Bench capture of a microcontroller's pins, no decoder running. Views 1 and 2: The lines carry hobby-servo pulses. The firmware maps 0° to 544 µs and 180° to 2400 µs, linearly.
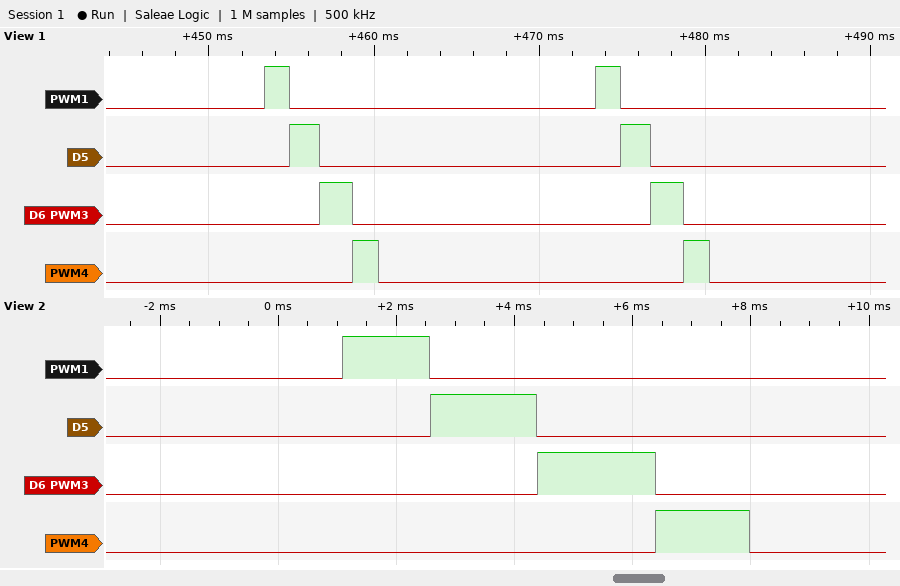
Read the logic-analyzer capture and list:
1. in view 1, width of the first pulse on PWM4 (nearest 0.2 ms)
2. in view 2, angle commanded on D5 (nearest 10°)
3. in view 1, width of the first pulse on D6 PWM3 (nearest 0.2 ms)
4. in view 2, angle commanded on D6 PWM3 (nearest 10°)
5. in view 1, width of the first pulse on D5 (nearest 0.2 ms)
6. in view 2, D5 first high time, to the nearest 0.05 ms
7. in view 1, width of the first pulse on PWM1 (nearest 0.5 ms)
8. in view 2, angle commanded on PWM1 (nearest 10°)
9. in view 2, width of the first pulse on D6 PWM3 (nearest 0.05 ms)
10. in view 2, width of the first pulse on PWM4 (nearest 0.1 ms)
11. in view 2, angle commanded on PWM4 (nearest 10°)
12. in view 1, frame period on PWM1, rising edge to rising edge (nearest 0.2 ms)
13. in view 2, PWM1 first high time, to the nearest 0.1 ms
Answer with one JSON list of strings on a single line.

["1.6 ms", "120°", "2.0 ms", "140°", "1.8 ms", "1.80 ms", "1.5 ms", "90°", "2.00 ms", "1.6 ms", "100°", "20.0 ms", "1.5 ms"]
